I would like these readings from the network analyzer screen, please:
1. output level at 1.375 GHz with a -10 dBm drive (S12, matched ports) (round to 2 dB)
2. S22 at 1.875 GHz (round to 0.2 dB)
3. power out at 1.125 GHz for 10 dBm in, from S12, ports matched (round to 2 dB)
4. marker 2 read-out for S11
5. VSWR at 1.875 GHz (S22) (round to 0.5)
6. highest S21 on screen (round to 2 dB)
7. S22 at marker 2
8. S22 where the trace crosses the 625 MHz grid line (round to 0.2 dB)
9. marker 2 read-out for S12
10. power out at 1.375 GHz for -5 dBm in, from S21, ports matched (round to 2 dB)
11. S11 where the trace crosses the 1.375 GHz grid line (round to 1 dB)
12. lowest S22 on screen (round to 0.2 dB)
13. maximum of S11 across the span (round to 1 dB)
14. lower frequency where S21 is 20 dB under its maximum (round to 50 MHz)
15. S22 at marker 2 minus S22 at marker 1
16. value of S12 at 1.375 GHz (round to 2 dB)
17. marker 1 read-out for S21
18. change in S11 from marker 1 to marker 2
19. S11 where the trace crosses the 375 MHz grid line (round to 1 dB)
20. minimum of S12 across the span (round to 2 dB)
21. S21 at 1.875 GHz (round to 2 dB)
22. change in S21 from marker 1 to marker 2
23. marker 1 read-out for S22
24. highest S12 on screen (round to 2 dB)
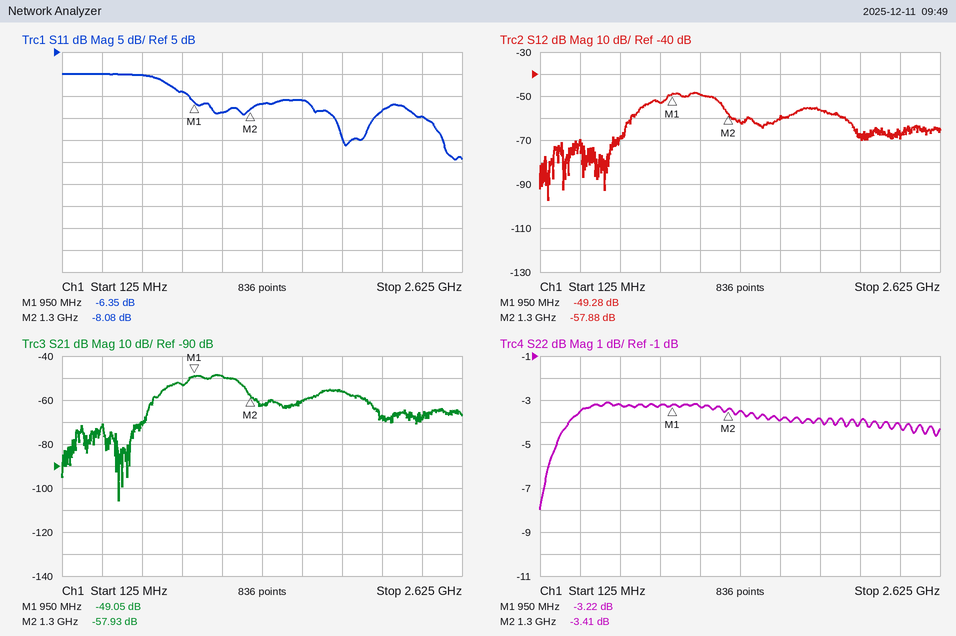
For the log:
-72 dBm
-3.8 dB
-40 dBm
-8.08 dB
4.5
-48 dB
-3.41 dB
-3.2 dB
-57.88 dB
-68 dBm
-7 dB
-8.0 dB
0 dB
650 MHz
-0.19 dB
-62 dB
-49.05 dB
-1.73 dB
0 dB
-98 dB
-56 dB
-8.88 dB
-3.22 dB
-48 dB
